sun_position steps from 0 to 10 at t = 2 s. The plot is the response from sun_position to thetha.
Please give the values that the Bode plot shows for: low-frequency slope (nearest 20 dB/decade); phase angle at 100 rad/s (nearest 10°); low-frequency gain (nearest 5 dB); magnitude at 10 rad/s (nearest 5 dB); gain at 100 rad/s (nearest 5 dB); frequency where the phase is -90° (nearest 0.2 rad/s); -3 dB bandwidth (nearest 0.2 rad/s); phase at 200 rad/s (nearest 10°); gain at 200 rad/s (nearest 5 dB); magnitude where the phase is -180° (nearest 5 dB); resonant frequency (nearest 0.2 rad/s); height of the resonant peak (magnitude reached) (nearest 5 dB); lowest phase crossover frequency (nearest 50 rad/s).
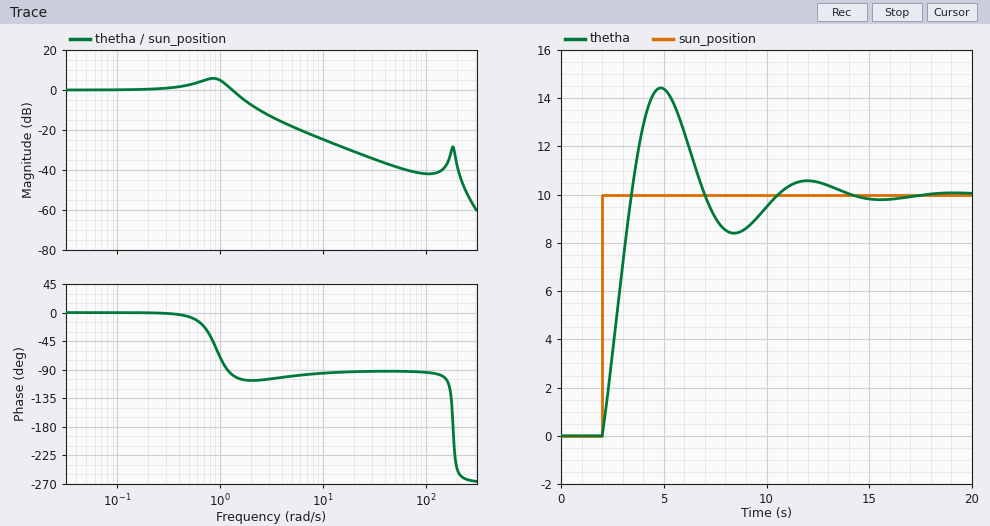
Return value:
0 dB/decade
-90°
0 dB
-25 dB
-40 dB
1.2 rad/s
1.6 rad/s
-240°
-35 dB
-30 dB
0.8 rad/s
5 dB
200 rad/s
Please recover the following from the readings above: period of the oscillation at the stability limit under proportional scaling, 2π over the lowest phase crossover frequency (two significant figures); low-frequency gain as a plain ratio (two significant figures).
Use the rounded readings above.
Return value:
0.031 s
1.0
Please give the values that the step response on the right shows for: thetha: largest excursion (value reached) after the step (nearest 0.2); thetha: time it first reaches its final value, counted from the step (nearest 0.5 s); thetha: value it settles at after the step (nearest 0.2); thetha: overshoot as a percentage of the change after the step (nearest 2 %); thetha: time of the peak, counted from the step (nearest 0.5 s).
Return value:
14.4
1.5 s
10.0
44 %
3.0 s
